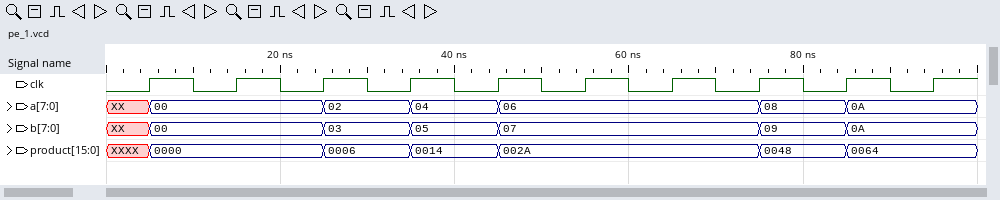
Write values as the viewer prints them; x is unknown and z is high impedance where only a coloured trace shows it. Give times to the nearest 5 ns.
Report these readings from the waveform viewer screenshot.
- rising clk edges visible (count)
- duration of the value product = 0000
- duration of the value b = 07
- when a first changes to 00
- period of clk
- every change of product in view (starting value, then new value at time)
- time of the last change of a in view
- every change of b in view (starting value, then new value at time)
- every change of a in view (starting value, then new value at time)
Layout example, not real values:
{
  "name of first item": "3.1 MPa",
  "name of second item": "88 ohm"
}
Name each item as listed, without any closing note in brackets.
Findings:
{
  "rising clk edges visible": "10",
  "duration of the value product = 0000": "20 ns",
  "duration of the value b = 07": "30 ns",
  "when a first changes to 00": "5 ns",
  "period of clk": "10 ns",
  "every change of product in view": "XXXX, 0000 at 5 ns, 0006 at 25 ns, 0014 at 35 ns, 002A at 45 ns, 0048 at 75 ns, 0064 at 85 ns",
  "time of the last change of a in view": "85 ns",
  "every change of b in view": "XX, 00 at 5 ns, 03 at 25 ns, 05 at 35 ns, 07 at 45 ns, 09 at 75 ns, 0A at 85 ns",
  "every change of a in view": "XX, 00 at 5 ns, 02 at 25 ns, 04 at 35 ns, 06 at 45 ns, 08 at 75 ns, 0A at 85 ns"
}
